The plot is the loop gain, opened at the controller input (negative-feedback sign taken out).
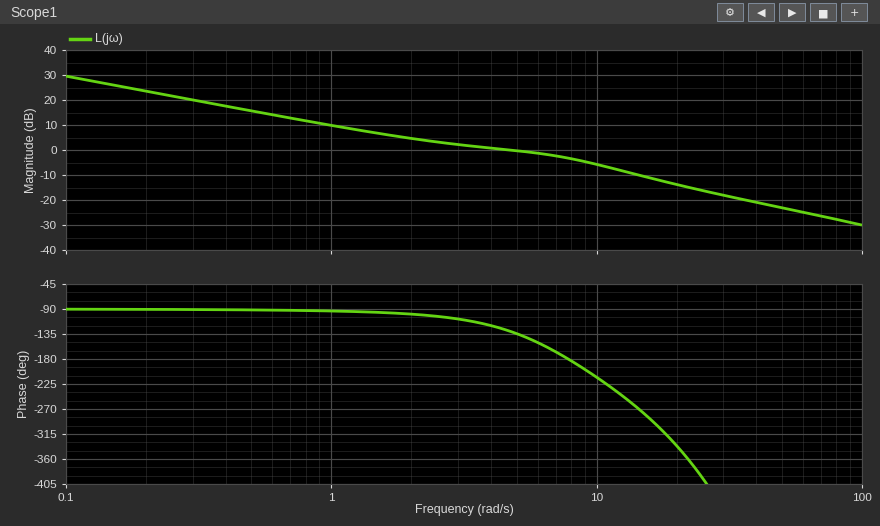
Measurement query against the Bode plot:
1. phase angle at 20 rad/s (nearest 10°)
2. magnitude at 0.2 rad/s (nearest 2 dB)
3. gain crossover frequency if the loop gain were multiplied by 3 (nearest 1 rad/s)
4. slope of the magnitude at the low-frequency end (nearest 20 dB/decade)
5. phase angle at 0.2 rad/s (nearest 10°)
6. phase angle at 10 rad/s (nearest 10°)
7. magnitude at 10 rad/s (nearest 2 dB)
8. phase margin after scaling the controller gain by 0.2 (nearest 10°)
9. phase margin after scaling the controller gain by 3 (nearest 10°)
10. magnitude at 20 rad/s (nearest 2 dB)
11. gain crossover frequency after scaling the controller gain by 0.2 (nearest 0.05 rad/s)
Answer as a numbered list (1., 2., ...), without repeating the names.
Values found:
1. -340°
2. 24 dB
3. 14 rad/s
4. -20 dB/decade
5. -90°
6. -210°
7. -6 dB
8. 90°
9. -80°
10. -14 dB
11. 0.60 rad/s
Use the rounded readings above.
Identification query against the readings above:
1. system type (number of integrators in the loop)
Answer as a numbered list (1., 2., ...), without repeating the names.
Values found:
1. 1
